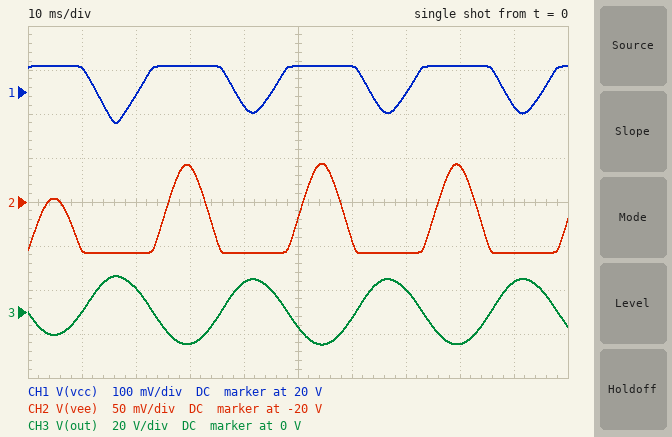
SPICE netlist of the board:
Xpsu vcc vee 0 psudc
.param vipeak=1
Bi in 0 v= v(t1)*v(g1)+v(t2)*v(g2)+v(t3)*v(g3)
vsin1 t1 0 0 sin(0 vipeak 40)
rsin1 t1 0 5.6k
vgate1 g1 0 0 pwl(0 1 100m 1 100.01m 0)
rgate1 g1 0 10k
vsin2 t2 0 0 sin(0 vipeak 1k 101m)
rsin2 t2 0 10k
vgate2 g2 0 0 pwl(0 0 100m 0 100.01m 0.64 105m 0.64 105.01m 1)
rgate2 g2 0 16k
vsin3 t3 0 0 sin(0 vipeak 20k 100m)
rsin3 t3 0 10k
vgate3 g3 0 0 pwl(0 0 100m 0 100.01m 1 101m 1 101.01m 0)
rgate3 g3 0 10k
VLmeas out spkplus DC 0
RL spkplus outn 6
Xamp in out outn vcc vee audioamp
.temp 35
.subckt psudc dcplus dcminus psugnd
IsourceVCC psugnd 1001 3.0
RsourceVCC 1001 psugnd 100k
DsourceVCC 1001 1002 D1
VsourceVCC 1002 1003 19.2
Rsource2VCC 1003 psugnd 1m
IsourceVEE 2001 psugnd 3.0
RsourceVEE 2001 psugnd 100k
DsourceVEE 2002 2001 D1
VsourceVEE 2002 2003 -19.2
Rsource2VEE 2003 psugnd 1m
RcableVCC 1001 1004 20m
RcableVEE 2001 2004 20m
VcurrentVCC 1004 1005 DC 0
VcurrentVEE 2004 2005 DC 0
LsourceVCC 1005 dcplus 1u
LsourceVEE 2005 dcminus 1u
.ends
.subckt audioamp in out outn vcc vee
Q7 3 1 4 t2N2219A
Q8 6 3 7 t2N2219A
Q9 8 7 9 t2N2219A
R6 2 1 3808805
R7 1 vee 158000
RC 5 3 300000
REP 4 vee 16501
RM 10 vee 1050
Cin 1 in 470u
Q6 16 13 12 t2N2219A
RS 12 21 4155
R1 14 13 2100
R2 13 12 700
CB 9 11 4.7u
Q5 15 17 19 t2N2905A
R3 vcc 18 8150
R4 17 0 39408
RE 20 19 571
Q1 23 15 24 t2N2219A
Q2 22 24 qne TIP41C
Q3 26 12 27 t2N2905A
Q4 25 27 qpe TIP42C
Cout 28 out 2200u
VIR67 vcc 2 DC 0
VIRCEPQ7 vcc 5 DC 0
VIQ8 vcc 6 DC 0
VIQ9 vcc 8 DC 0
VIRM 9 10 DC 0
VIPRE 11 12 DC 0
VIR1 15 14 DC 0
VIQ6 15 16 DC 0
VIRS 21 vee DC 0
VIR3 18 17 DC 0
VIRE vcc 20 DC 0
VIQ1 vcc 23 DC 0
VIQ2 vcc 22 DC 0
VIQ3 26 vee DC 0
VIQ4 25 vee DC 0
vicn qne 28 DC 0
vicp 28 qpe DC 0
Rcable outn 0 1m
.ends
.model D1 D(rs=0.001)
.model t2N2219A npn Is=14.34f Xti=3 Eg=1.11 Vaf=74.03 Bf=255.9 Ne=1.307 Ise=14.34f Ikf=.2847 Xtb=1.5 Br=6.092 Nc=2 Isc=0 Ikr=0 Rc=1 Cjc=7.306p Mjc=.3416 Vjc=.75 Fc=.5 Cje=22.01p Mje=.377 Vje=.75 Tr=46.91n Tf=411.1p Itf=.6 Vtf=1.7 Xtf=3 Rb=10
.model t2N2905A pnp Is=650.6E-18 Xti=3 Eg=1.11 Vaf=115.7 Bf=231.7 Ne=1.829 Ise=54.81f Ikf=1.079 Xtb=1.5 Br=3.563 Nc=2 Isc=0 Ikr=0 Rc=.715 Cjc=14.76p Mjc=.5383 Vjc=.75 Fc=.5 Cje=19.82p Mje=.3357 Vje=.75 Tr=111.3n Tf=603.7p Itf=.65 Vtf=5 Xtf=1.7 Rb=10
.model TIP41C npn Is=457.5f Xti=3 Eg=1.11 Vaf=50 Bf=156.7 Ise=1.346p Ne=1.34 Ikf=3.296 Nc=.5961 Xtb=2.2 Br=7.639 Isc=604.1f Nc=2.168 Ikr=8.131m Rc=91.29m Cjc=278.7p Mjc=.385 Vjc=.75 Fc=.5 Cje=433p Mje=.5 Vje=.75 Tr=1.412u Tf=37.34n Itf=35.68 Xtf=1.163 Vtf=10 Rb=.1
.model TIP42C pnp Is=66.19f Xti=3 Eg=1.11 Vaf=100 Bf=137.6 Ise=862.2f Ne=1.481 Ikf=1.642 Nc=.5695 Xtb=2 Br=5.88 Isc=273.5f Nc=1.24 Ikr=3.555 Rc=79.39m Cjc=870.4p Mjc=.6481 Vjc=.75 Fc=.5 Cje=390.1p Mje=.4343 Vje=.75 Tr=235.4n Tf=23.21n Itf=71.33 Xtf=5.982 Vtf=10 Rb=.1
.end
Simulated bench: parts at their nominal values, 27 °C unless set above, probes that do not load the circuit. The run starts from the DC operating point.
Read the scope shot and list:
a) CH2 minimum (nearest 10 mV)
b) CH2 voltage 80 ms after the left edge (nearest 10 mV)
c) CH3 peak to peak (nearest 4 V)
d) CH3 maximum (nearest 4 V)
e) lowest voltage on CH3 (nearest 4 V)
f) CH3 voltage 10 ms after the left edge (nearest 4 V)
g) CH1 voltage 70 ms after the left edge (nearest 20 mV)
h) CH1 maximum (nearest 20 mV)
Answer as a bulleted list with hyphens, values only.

- -20.06 V
- -19.96 V
- 32 V
- 16 V
- -16 V
- 0 V
- 20.00 V
- 20.06 V
